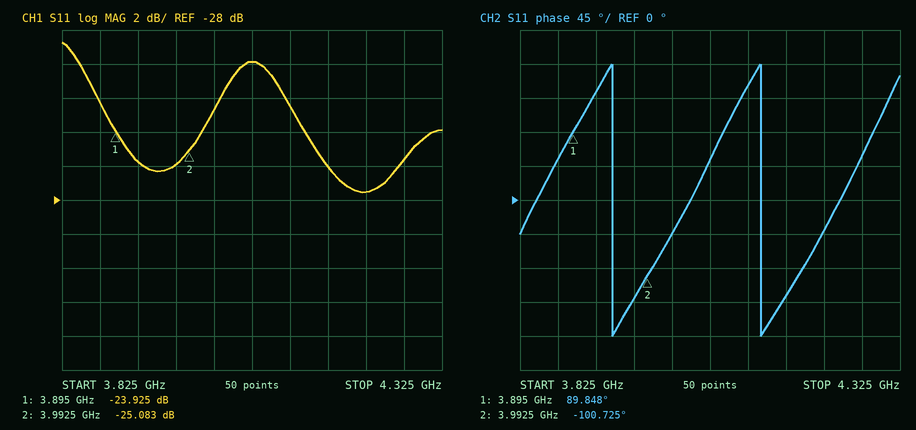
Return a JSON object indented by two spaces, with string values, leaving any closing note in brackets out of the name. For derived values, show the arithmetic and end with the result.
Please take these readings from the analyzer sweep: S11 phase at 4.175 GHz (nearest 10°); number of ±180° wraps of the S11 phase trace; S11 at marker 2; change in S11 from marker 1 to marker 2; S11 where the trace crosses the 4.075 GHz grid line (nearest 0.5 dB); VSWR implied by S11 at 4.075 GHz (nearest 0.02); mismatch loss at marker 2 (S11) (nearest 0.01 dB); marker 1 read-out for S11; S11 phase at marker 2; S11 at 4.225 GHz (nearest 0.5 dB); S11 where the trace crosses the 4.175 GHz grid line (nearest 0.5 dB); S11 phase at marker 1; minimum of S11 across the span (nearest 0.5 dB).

{
  "S11 phase at 4.175 GHz": "-130°",
  "number of ±180° wraps of the S11 phase trace": "2",
  "S11 at marker 2": "-25.083 dB",
  "change in S11 from marker 1 to marker 2": "-25.083 − (-23.925) = -1.158 dB",
  "S11 where the trace crosses the 4.075 GHz grid line": "-20.0 dB",
  "VSWR implied by S11 at 4.075 GHz": "|Γ| = 10^(-20/20) = 0.1000; VSWR = (1 + 0.1000)/(1 − 0.1000) ≈ 1.22",
  "mismatch loss at marker 2 (S11)": "−10 log10(1 − 10^(-25.083/10)) ≈ 0.01 dB",
  "marker 1 read-out for S11": "-23.925 dB",
  "S11 phase at marker 2": "-100.725°",
  "S11 at 4.225 GHz": "-27.5 dB",
  "S11 where the trace crosses the 4.175 GHz grid line": "-26.0 dB",
  "S11 phase at marker 1": "89.848°",
  "minimum of S11 across the span": "-27.5 dB"
}
